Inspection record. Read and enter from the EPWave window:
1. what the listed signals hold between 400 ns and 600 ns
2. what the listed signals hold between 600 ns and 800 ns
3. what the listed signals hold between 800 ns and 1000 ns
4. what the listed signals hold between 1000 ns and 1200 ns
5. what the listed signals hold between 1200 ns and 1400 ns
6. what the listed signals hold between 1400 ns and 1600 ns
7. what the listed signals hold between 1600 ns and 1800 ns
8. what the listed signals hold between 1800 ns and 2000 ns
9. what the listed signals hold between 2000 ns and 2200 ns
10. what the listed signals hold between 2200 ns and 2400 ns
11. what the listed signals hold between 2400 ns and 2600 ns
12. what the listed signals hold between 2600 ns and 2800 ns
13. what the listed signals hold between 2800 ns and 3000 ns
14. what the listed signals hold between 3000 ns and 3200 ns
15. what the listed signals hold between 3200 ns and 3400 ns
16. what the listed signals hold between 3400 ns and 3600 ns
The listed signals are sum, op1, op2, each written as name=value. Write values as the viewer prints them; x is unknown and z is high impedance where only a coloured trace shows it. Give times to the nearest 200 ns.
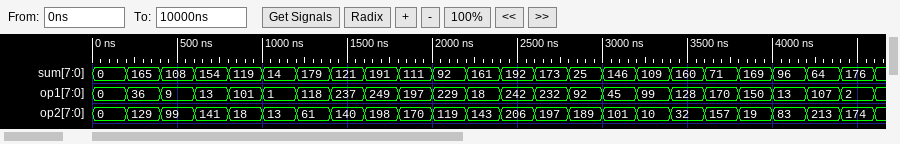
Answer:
sum=108, op1=9, op2=99
sum=154, op1=13, op2=141
sum=119, op1=101, op2=18
sum=14, op1=1, op2=13
sum=179, op1=118, op2=61
sum=121, op1=237, op2=140
sum=191, op1=249, op2=198
sum=111, op1=197, op2=170
sum=92, op1=229, op2=119
sum=161, op1=18, op2=143
sum=192, op1=242, op2=206
sum=173, op1=232, op2=197
sum=25, op1=92, op2=189
sum=146, op1=45, op2=101
sum=109, op1=99, op2=10
sum=160, op1=128, op2=32
